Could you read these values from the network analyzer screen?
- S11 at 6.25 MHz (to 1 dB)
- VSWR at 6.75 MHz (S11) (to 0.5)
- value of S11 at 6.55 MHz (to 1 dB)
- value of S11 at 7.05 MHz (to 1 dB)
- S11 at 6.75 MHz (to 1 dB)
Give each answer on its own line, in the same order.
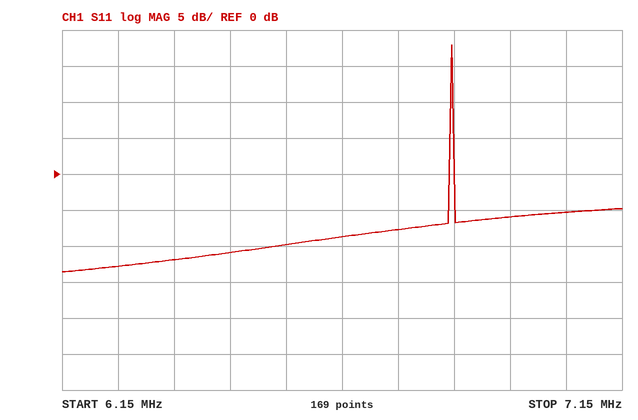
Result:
-13 dB
2.5
-10 dB
-5 dB
-8 dB
